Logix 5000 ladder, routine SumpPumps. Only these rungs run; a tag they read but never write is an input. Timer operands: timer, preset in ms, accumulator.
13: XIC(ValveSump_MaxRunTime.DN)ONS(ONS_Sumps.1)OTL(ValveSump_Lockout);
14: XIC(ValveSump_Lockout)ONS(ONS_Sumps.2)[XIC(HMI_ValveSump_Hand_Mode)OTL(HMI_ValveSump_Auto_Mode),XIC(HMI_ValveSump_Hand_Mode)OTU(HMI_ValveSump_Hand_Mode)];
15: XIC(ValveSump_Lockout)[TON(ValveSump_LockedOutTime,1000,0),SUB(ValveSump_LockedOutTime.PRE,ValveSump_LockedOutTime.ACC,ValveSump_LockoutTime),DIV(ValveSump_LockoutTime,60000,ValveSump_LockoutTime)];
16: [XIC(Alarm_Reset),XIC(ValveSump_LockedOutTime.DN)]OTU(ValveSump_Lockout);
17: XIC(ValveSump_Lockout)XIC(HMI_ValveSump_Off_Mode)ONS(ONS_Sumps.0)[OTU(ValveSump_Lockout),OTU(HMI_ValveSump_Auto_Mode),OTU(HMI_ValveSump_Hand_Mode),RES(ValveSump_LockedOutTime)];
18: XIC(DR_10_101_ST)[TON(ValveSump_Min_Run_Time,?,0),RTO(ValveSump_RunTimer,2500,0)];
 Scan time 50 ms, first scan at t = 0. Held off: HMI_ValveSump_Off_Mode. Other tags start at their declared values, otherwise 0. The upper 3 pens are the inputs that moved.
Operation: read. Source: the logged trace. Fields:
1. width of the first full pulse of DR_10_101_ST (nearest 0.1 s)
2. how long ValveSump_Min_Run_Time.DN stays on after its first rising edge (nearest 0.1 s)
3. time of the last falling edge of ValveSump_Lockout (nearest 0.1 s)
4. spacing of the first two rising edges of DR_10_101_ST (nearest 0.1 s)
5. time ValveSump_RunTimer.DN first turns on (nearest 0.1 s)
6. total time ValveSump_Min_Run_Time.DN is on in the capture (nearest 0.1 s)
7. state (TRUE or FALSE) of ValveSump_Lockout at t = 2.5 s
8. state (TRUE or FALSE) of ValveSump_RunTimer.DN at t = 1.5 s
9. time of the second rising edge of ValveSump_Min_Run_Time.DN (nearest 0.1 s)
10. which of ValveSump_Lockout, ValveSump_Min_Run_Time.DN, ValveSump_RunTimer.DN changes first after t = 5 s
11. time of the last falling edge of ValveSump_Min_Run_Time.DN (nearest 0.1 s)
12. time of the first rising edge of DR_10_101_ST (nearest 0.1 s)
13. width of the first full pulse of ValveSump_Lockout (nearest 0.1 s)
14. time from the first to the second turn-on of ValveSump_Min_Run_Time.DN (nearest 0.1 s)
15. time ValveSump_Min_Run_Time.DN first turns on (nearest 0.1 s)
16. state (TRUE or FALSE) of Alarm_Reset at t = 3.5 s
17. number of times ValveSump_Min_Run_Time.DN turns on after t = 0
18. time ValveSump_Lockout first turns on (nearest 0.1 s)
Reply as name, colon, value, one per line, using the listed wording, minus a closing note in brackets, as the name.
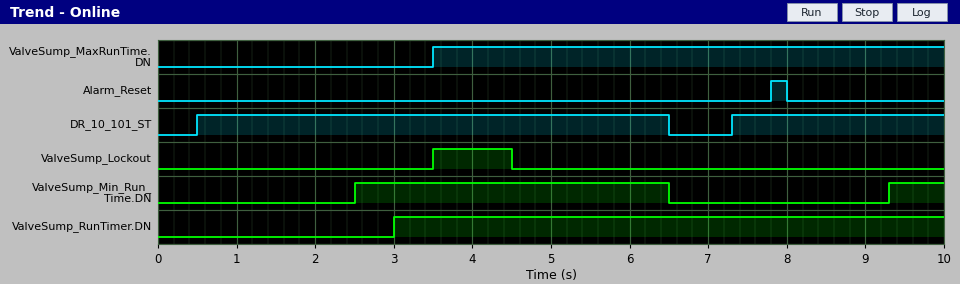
width of the first full pulse of DR_10_101_ST: 6.0 s
how long ValveSump_Min_Run_Time.DN stays on after its first rising edge: 4.0 s
time of the last falling edge of ValveSump_Lockout: 4.5 s
spacing of the first two rising edges of DR_10_101_ST: 6.8 s
time ValveSump_RunTimer.DN first turns on: 3.0 s
total time ValveSump_Min_Run_Time.DN is on in the capture: 4.7 s
state (TRUE or FALSE) of ValveSump_Lockout at t = 2.5 s: FALSE
state (TRUE or FALSE) of ValveSump_RunTimer.DN at t = 1.5 s: FALSE
time of the second rising edge of ValveSump_Min_Run_Time.DN: 9.3 s
which of ValveSump_Lockout, ValveSump_Min_Run_Time.DN, ValveSump_RunTimer.DN changes first after t = 5 s: ValveSump_Min_Run_Time.DN
time of the last falling edge of ValveSump_Min_Run_Time.DN: 6.5 s
time of the first rising edge of DR_10_101_ST: 0.5 s
width of the first full pulse of ValveSump_Lockout: 1.0 s
time from the first to the second turn-on of ValveSump_Min_Run_Time.DN: 6.8 s
time ValveSump_Min_Run_Time.DN first turns on: 2.5 s
state (TRUE or FALSE) of Alarm_Reset at t = 3.5 s: FALSE
number of times ValveSump_Min_Run_Time.DN turns on after t = 0: 2
time ValveSump_Lockout first turns on: 3.5 s
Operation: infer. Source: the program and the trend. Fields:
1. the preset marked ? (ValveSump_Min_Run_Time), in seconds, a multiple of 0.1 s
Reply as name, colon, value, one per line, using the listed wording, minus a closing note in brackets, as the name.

the preset marked ? (ValveSump_Min_Run_Time), in seconds, a multiple of 0.1 s: 2.0 s
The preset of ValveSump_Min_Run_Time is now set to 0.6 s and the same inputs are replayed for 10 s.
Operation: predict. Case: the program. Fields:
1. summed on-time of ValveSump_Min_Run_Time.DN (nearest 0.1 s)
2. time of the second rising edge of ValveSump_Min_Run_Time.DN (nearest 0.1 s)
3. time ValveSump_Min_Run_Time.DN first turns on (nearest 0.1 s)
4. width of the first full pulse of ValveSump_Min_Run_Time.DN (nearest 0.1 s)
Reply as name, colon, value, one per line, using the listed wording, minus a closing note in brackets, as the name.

summed on-time of ValveSump_Min_Run_Time.DN: 7.5 s
time of the second rising edge of ValveSump_Min_Run_Time.DN: 7.9 s
time ValveSump_Min_Run_Time.DN first turns on: 1.1 s
width of the first full pulse of ValveSump_Min_Run_Time.DN: 5.4 s
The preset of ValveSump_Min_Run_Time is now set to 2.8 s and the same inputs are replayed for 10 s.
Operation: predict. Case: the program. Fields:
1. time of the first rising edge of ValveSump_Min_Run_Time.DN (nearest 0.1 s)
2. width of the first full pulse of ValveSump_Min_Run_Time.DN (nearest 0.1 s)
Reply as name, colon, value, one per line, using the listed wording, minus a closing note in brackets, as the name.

time of the first rising edge of ValveSump_Min_Run_Time.DN: 3.3 s
width of the first full pulse of ValveSump_Min_Run_Time.DN: 3.2 s
